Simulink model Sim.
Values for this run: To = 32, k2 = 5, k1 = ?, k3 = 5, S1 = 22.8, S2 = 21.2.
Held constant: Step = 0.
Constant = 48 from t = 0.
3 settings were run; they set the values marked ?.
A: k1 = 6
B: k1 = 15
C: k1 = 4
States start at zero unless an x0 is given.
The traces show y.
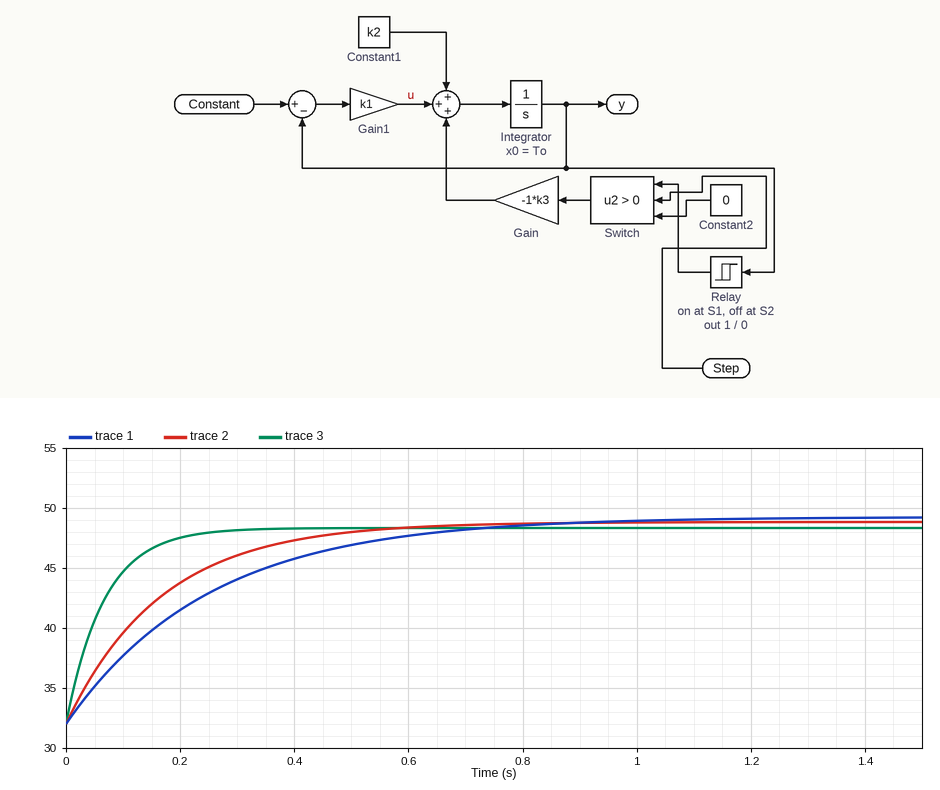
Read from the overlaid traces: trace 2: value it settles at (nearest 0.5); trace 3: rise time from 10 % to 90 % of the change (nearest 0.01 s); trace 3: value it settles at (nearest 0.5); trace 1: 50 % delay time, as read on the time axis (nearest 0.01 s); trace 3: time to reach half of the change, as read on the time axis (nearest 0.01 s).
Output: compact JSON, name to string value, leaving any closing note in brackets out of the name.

{"trace 2: value it settles at": "49.0", "trace 3: rise time from 10 % to 90 % of the change": "0.15 s", "trace 3: value it settles at": "48.5", "trace 1: 50 % delay time, as read on the time axis": "0.17 s", "trace 3: time to reach half of the change, as read on the time axis": "0.05 s"}
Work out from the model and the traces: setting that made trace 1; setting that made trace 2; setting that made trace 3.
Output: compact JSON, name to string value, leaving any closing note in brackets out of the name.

{"setting that made trace 1": "C", "setting that made trace 2": "A", "setting that made trace 3": "B"}
